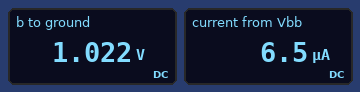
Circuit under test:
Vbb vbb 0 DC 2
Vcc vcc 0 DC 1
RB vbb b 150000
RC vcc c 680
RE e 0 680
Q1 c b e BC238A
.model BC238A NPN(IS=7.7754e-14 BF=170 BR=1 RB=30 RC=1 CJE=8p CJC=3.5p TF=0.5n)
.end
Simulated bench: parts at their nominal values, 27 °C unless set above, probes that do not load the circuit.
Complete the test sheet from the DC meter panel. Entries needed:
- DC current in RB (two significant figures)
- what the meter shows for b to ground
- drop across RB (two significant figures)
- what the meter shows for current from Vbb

6.5 µA
1.022 V
980 mV
6.5 µA
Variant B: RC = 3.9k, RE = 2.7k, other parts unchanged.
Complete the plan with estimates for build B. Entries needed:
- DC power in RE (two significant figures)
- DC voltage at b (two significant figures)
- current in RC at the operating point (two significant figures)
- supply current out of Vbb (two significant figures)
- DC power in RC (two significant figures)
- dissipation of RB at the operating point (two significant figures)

55 µW
940 mV
140 µA
7.1 µA
72 µW
7.5 µW
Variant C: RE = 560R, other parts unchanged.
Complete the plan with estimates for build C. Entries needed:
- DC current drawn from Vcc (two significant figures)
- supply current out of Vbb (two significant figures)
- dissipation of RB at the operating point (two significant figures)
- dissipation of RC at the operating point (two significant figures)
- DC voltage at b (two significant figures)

690 µA
6.8 µA
6.9 µW
320 µW
980 mV
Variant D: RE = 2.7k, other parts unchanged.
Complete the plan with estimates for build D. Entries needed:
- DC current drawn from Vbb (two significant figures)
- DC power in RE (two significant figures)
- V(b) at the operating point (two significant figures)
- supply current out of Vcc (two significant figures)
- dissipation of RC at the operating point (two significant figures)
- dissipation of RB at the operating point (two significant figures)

4.8 µA
190 µW
1.3 V
260 µA
45 µW
3.5 µW
